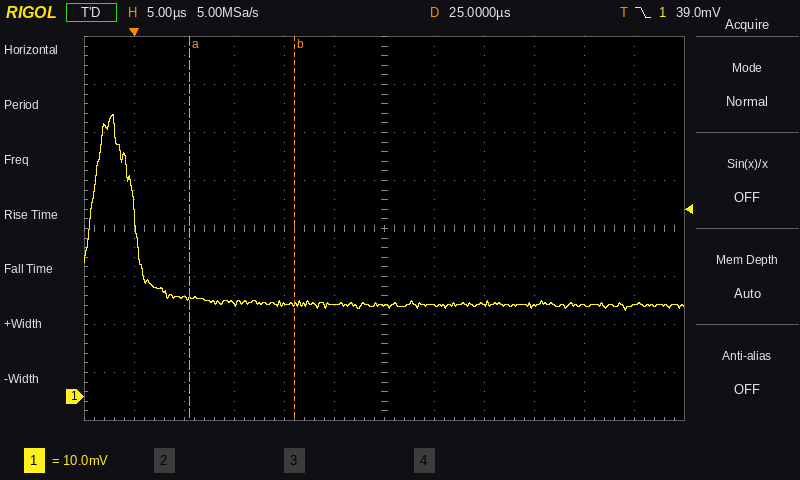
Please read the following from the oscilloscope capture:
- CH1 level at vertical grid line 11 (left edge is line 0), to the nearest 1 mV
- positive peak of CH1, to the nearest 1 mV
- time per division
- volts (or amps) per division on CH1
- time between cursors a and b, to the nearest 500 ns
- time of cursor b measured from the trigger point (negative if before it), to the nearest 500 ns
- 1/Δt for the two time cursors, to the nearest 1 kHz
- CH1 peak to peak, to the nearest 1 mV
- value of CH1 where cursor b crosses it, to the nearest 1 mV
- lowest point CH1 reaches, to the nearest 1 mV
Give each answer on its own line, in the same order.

19 mV
59 mV
5 µs
10 mV
10.5 µs
+16.0 µs
95 kHz
41 mV
19 mV
18 mV
